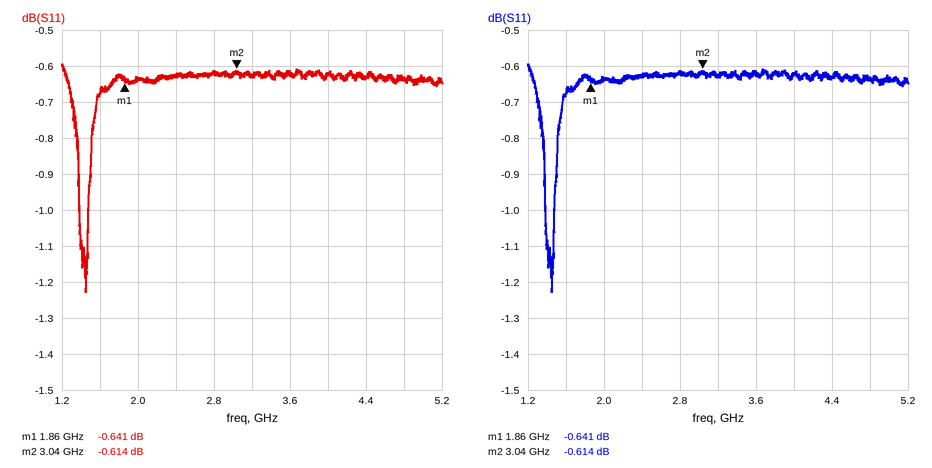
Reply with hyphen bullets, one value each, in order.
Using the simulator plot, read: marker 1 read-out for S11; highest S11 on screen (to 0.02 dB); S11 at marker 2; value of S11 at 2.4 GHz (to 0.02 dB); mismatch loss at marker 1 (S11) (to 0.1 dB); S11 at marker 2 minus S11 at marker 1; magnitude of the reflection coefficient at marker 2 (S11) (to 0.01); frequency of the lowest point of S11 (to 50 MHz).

- -0.641 dB
- -0.60 dB
- -0.614 dB
- -0.62 dB
- 8.6 dB
- 0.027 dB
- 0.93
- 1.45 GHz
